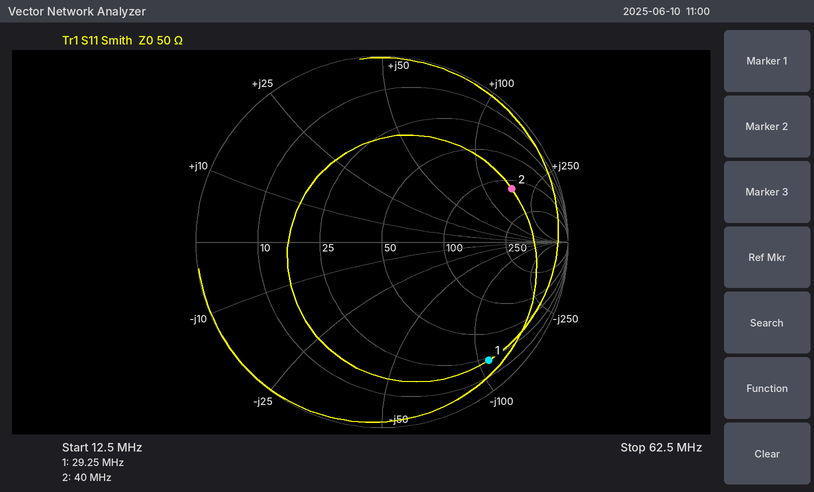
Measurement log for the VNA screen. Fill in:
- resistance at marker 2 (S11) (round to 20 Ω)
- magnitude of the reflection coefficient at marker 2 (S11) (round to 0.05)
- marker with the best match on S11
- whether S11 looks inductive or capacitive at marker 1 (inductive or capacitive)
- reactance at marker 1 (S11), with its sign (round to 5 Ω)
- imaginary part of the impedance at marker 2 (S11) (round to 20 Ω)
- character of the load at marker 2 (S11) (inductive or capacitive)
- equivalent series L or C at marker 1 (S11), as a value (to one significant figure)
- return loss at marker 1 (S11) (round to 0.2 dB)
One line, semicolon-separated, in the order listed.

120 Ω; 0.75; marker 2; capacitive; -110 Ω; +160 Ω; inductive; 50 pF; 1.4 dB
